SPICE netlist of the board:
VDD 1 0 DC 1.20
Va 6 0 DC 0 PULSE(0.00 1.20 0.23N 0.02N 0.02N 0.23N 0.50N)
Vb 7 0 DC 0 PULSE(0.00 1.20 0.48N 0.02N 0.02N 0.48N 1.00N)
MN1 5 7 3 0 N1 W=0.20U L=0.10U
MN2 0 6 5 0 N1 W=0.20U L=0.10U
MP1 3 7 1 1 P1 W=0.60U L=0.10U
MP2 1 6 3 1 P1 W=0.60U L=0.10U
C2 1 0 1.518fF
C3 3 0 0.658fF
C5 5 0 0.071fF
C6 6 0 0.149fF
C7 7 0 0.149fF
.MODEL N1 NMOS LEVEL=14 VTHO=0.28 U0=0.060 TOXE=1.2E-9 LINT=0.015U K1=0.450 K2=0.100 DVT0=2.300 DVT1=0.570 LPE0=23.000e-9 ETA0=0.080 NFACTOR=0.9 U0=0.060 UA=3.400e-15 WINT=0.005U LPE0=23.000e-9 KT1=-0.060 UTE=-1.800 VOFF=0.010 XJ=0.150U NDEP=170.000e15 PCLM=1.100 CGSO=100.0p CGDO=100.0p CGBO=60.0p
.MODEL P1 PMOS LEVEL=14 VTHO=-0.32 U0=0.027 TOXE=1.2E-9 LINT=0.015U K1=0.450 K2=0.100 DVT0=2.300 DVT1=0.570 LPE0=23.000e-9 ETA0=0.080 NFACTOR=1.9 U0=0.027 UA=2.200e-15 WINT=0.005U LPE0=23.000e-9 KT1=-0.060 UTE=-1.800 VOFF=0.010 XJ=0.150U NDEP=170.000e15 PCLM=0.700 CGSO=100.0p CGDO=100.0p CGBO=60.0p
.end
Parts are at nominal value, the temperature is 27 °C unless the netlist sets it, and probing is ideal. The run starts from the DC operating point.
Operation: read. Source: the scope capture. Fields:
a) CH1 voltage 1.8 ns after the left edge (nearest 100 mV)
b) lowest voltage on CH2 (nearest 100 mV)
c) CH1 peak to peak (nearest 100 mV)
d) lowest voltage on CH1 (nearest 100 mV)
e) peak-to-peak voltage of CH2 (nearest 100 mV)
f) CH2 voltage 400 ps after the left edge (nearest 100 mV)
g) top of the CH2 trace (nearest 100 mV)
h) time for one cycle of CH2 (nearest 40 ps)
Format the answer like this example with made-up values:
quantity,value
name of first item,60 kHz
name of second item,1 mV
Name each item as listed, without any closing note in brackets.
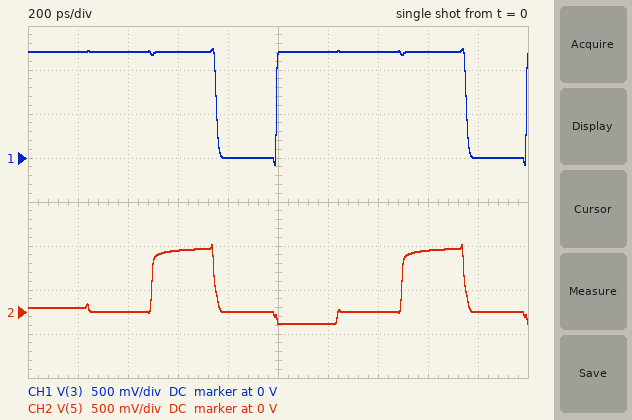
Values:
quantity,value
CH1 voltage 1.8 ns after the left edge,0 V
lowest voltage on CH2,-100 mV
CH1 peak to peak,1.3 V
lowest voltage on CH1,-100 mV
peak-to-peak voltage of CH2,900 mV
CH2 voltage 400 ps after the left edge,0 V
top of the CH2 trace,800 mV
time for one cycle of CH2,1.00 ns
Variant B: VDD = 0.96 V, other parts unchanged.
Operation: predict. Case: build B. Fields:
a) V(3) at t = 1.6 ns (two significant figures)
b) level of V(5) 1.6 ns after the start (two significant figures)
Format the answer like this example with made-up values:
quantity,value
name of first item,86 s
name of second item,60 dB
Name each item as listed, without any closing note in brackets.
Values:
quantity,value
V(3) at t = 1.6 ns,960 mV
level of V(5) 1.6 ns after the start,680 mV
